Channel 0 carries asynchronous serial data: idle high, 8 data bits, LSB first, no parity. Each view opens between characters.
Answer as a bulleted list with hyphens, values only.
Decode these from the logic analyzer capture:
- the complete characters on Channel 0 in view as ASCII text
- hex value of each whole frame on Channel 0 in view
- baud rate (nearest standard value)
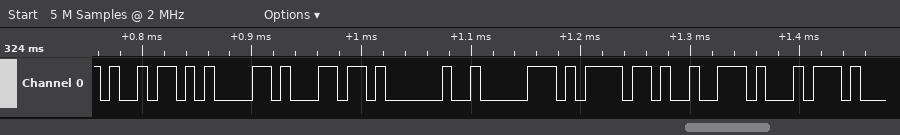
- "ial port"
- 69, 61, 6C, 20, 70, 6F, 72, 74
- 115200 baud
